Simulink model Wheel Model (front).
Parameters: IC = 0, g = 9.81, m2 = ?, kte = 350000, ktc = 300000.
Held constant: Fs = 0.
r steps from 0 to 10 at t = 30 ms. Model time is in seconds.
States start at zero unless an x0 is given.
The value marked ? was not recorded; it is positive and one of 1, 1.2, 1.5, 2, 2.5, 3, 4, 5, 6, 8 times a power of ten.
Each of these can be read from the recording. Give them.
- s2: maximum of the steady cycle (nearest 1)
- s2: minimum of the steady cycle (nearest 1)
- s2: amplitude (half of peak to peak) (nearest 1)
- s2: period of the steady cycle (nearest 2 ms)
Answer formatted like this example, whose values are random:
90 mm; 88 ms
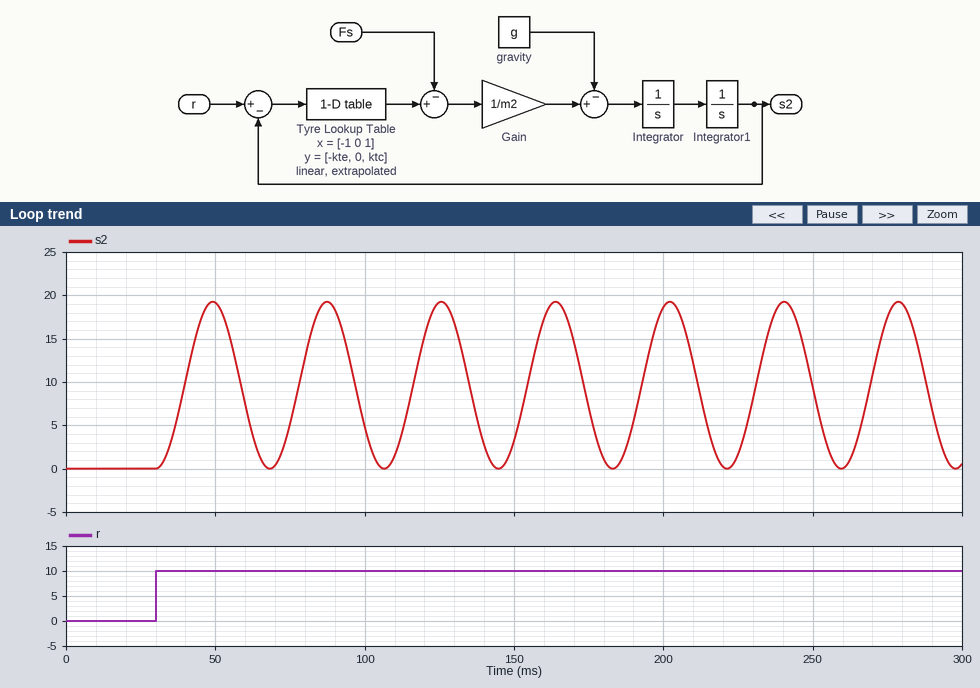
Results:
19; 0; 10; 38 ms
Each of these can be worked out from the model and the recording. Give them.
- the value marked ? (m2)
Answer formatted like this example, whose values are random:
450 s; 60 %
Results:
12
